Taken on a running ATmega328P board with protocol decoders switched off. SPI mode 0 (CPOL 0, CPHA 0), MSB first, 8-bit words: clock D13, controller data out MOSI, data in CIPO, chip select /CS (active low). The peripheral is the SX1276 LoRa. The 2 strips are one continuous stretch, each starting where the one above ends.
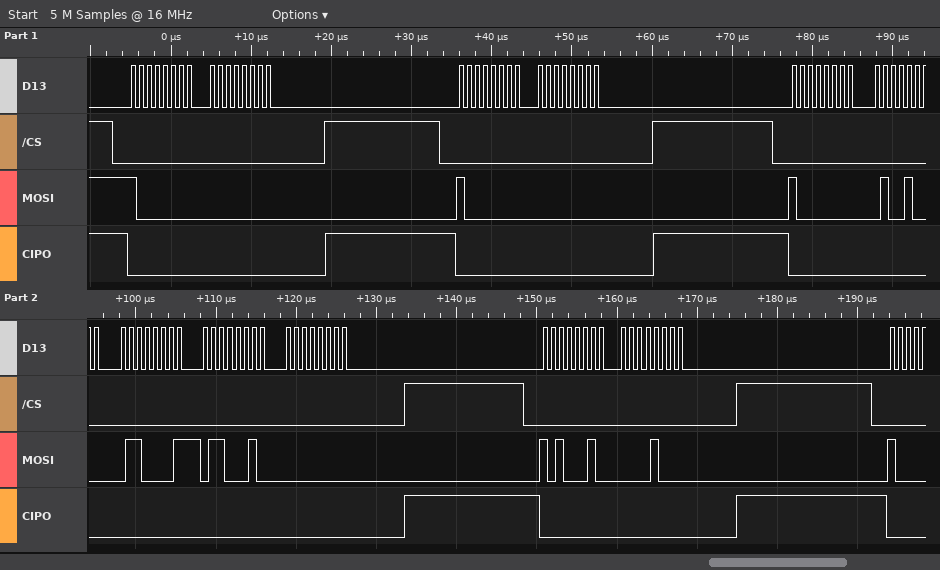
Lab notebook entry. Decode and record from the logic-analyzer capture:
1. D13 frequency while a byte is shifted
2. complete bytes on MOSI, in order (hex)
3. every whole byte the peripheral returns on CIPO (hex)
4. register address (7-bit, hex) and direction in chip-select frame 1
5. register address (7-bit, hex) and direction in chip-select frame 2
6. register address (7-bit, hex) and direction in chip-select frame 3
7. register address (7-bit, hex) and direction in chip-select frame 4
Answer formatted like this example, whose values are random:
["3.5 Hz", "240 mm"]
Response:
["1 MHz", "80 00 80 00 80 48 61 62 00 A2 08", "00 00 00 00 00 00 00 00 00 00 00", "0x00 write", "0x00 write", "0x00 write", "0x22 write"]
